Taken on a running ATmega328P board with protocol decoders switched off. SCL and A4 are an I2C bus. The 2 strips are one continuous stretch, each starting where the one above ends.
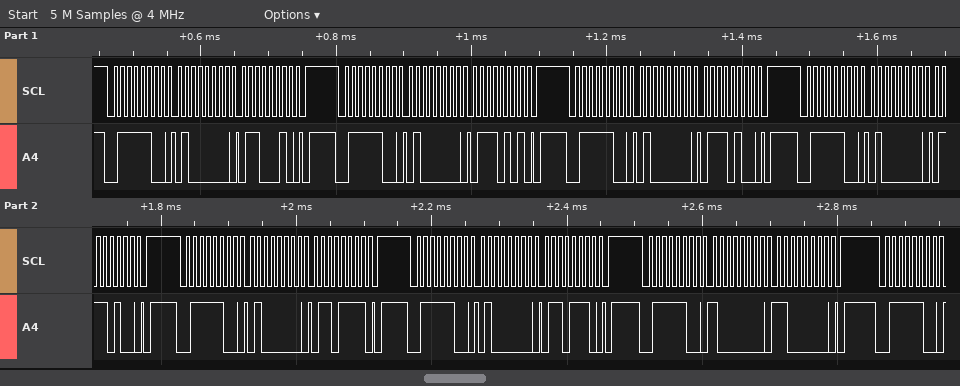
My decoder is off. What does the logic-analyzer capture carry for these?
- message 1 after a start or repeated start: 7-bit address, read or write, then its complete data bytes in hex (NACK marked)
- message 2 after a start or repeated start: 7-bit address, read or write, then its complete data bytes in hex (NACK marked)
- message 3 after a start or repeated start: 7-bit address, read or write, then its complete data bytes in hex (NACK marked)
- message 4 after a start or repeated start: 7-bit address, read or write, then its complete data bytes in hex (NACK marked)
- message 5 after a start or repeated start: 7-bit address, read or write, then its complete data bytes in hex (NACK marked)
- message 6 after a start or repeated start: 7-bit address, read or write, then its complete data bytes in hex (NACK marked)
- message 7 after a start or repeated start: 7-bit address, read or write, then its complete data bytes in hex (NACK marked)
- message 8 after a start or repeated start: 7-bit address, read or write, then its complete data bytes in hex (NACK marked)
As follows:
0x3E write: 40 62
0x3E write: 40 75
0x3E write: 40 74
0x3E write: 40 74
0x3E write: 40 6F
0x3E write: 40 6E
0x3E write: 80 C0
0x3E write
